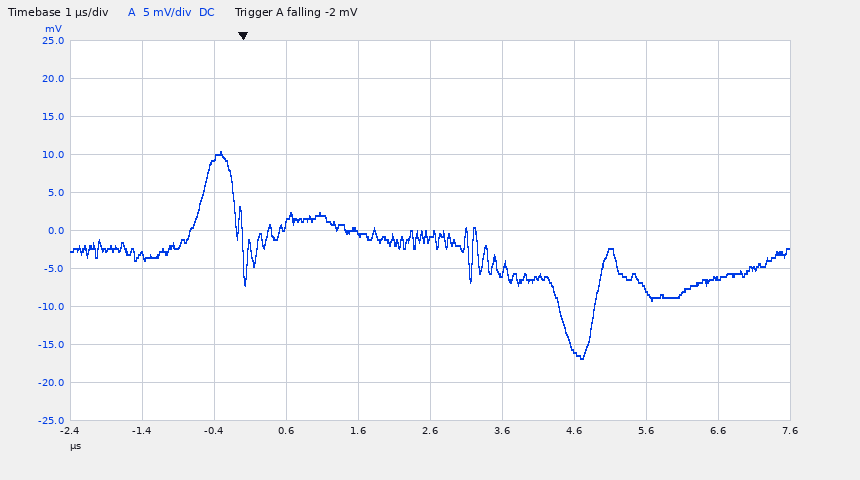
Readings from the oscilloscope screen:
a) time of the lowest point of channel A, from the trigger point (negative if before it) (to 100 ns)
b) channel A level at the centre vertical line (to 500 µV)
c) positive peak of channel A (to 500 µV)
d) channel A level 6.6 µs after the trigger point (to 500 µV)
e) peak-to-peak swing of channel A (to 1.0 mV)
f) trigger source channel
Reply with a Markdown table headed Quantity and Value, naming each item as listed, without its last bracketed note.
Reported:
| Quantity | Value |
|---|---|
| time of the lowest point of channel A, from the trigger point (negative if before it) | +4.7 µs |
| channel A level at the centre vertical line | -1.0 mV |
| positive peak of channel A | 10.5 mV |
| channel A level 6.6 µs after the trigger point | -6.0 mV |
| peak-to-peak swing of channel A | 27.0 mV |
| trigger source channel | channel A |
